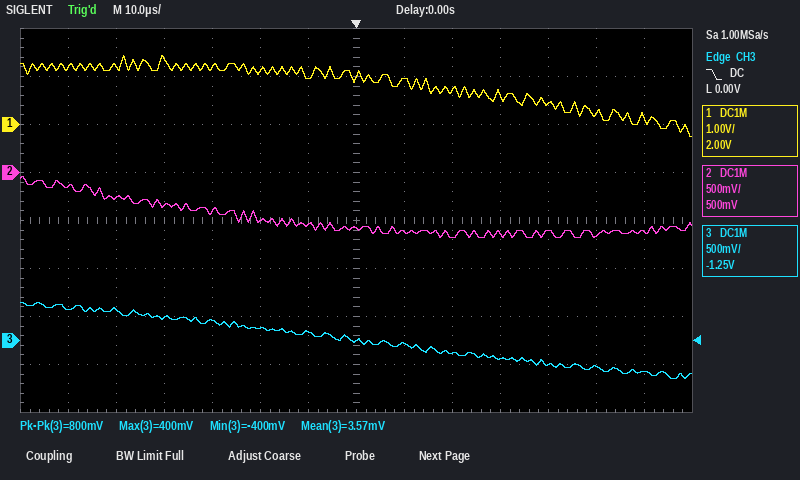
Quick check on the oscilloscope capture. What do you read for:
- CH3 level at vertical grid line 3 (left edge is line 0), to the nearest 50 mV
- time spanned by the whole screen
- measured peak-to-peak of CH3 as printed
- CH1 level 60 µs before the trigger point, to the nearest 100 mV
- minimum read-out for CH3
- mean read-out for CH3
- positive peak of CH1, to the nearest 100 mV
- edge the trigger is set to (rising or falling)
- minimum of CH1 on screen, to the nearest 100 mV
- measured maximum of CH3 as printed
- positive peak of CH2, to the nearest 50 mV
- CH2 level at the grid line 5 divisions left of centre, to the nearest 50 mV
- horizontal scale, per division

250 mV
140 µs
800 mV
1.2 V
-400 mV
3.57 mV
1.4 V
falling
-200 mV
400 mV
-50 mV
-250 mV
10 µs
